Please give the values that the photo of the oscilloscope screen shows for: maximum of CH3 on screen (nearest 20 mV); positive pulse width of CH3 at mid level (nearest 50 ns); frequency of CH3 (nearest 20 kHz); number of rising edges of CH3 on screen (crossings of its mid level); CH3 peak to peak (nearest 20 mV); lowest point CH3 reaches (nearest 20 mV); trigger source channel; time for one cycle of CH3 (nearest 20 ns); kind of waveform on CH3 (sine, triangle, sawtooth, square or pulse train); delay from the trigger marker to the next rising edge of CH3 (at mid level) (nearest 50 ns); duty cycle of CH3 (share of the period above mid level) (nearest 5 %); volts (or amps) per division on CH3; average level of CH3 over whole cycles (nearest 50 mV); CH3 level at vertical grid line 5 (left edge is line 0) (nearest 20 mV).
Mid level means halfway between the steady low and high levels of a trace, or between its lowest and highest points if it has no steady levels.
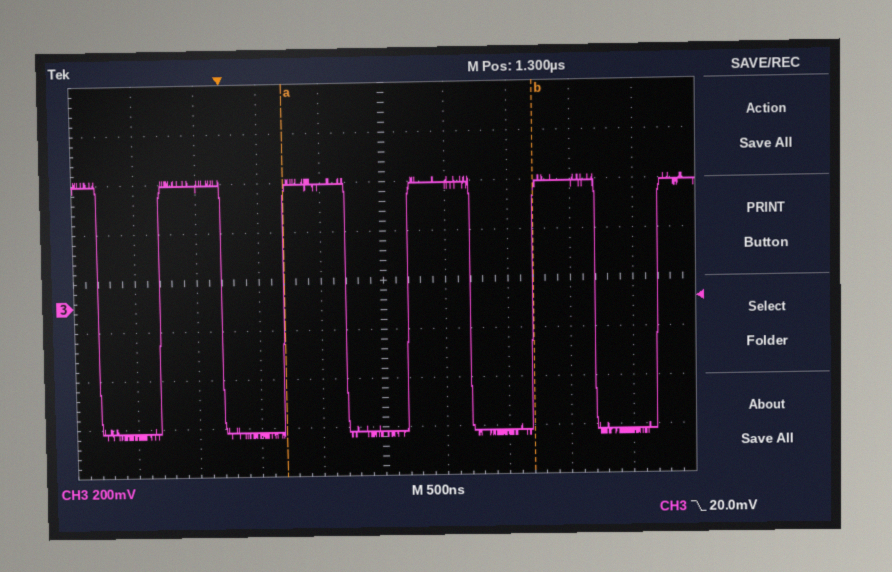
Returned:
520 mV
500 ns
1.00 MHz
5
1.06 V
-540 mV
CH3
1.00 µs
square
500 ns
50 %
200 mV
0 mV
-520 mV
